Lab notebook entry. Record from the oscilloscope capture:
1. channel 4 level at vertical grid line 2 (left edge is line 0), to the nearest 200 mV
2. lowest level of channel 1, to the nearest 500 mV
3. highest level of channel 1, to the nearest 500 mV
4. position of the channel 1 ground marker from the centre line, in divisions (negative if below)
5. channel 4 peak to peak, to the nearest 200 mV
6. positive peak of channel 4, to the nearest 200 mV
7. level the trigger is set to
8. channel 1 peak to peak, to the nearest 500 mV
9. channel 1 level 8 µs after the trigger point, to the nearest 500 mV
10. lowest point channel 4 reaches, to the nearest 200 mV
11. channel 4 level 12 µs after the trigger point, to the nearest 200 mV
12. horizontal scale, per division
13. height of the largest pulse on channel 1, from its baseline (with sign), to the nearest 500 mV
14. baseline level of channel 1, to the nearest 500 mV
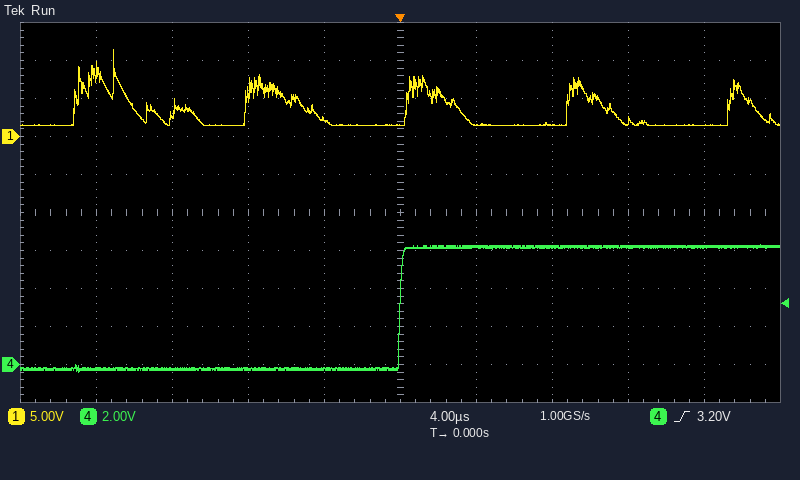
-200 mV
1.5 V
11.5 V
+2.0 div
6.8 V
6.4 V
3.20 V
10.0 V
1.5 V
-400 mV
6.2 V
4 µs
+10.0 V
1.5 V
